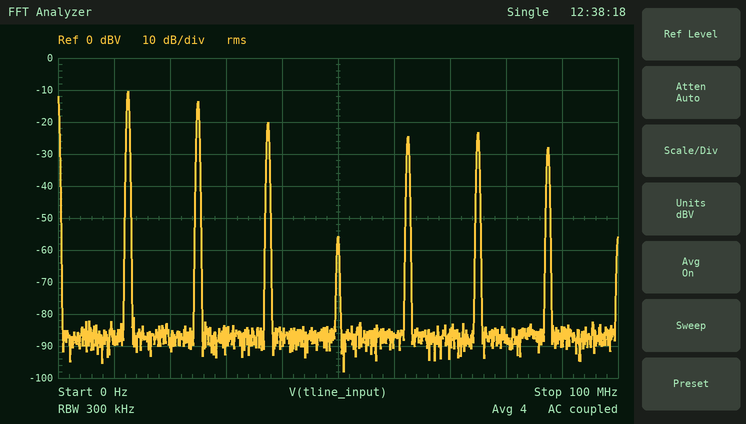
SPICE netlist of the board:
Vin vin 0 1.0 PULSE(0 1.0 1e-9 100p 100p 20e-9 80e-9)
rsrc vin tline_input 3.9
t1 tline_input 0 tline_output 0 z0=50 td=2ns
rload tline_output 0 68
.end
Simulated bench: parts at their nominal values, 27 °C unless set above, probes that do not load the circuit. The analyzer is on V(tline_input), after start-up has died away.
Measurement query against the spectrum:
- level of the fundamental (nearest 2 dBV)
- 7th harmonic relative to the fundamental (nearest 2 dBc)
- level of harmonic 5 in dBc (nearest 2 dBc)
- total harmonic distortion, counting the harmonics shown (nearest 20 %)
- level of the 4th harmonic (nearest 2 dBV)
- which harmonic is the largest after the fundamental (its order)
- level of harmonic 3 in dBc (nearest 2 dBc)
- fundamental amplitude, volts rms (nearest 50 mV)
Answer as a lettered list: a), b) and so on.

a) -10 dBV
b) -18 dBc
c) -14 dBc
d) 80 %
e) -56 dBV
f) 2
g) -10 dBc
h) 300 mV
